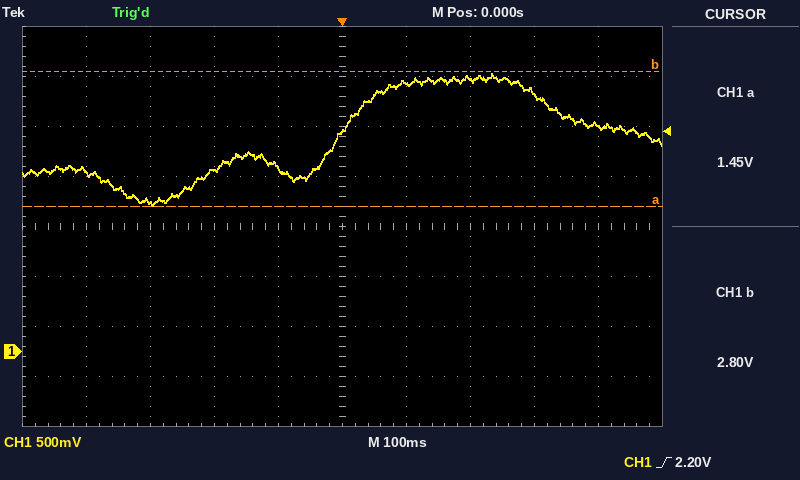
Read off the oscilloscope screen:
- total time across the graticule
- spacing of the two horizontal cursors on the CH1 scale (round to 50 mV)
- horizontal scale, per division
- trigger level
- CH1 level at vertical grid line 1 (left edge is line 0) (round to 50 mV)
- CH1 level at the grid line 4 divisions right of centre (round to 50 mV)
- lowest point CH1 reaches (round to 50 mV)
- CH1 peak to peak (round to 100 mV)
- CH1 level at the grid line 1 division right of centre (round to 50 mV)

1 s
1.35 V
100 ms
2.20 V
1.80 V
2.25 V
1.45 V
1.30 V
2.70 V
